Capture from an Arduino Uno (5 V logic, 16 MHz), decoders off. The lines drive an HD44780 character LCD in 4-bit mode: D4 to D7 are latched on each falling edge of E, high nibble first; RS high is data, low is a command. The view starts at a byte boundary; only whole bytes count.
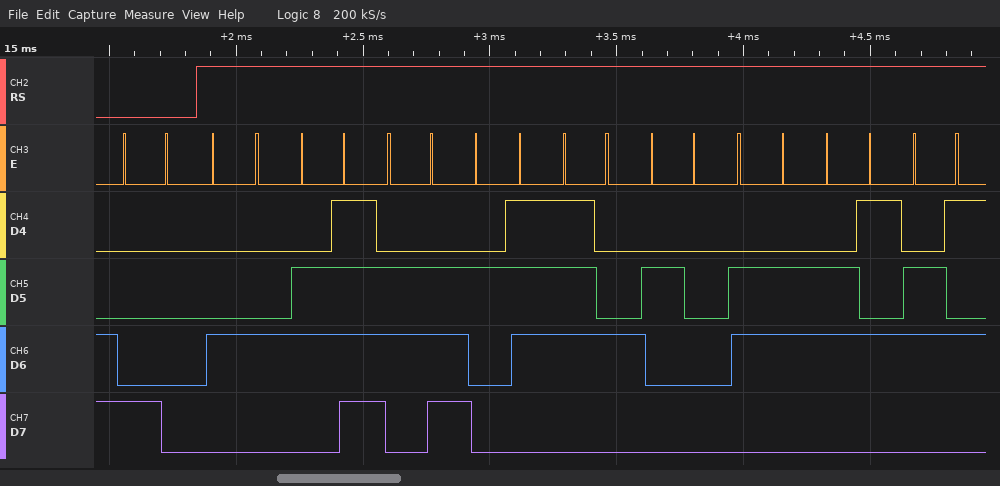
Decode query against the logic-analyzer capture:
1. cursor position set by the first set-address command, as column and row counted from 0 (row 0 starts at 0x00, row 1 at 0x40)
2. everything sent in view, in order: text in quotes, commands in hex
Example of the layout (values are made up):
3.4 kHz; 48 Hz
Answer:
column 0, row 0; 0x80 "Don't fee"
